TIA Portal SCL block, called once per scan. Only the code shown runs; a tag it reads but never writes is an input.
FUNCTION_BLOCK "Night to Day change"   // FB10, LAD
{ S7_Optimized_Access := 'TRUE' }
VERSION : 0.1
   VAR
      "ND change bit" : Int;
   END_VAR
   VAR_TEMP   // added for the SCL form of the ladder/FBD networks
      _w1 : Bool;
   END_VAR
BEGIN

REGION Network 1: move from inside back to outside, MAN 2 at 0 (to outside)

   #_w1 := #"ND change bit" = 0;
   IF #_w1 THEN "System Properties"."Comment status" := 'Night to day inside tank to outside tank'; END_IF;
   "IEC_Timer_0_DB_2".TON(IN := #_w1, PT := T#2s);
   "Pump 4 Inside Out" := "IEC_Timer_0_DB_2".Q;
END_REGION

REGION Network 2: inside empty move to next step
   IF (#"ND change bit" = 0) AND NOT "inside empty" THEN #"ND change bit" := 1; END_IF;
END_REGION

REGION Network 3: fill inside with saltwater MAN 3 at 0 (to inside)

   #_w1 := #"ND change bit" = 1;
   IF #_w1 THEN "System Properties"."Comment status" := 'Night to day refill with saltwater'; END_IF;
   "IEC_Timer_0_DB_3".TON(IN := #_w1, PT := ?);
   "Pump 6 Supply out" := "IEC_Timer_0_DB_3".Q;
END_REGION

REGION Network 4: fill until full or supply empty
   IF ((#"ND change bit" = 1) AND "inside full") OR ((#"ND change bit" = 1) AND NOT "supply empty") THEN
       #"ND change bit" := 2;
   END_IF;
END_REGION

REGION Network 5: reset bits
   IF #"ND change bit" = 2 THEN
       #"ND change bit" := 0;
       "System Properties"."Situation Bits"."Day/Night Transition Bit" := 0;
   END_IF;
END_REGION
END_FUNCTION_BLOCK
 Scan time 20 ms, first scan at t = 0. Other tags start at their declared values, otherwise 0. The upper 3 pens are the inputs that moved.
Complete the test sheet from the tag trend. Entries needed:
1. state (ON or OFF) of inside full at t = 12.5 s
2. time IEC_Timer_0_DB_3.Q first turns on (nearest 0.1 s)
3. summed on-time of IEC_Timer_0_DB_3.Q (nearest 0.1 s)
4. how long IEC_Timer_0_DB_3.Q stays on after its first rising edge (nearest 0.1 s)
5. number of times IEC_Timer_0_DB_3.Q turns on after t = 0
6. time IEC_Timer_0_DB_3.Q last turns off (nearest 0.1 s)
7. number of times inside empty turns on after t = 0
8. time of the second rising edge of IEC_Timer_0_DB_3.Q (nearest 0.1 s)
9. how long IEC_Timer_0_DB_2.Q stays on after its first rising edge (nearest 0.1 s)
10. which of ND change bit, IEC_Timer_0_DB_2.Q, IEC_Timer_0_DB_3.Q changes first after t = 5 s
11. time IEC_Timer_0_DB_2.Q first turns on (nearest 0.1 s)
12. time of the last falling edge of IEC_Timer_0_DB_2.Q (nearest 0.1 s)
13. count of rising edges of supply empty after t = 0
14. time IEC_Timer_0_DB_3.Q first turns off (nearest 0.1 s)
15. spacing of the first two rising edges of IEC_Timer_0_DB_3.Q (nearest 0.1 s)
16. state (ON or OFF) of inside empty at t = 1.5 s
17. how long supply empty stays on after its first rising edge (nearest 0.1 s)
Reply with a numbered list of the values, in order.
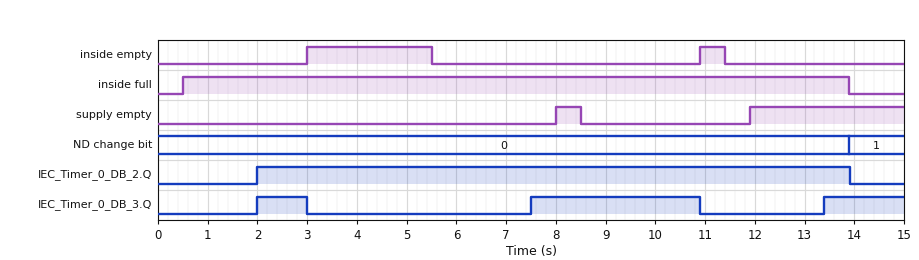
1. ON
2. 2.0 s
3. 6.0 s
4. 1.0 s
5. 3
6. 10.9 s
7. 2
8. 7.5 s
9. 11.9 s
10. IEC_Timer_0_DB_3.Q
11. 2.0 s
12. 13.9 s
13. 2
14. 3.0 s
15. 5.5 s
16. OFF
17. 0.5 s
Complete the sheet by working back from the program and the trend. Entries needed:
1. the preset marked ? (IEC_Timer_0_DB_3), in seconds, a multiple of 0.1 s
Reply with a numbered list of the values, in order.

1. 2.0 s
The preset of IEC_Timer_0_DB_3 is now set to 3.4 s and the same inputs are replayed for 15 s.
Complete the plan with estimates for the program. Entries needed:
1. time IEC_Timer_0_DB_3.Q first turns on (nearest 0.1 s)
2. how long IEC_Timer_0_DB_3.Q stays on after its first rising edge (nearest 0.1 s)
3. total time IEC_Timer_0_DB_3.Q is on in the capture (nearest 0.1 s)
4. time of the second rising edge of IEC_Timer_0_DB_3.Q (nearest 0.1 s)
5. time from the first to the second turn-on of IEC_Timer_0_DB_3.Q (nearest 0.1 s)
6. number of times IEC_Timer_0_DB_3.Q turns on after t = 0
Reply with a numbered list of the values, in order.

1. 8.9 s
2. 2.0 s
3. 2.2 s
4. 14.8 s
5. 5.9 s
6. 2
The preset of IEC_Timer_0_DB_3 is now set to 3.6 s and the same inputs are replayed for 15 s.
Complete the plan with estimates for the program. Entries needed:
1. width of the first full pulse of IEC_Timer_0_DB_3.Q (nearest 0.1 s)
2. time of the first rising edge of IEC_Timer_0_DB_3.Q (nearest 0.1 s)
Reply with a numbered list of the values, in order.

1. 1.8 s
2. 9.1 s
